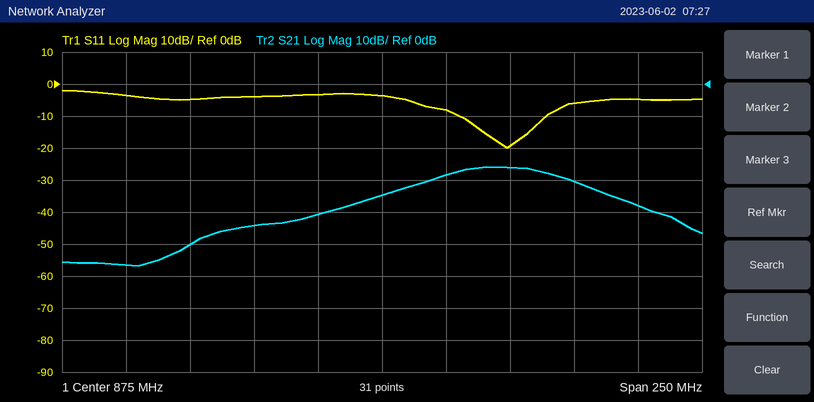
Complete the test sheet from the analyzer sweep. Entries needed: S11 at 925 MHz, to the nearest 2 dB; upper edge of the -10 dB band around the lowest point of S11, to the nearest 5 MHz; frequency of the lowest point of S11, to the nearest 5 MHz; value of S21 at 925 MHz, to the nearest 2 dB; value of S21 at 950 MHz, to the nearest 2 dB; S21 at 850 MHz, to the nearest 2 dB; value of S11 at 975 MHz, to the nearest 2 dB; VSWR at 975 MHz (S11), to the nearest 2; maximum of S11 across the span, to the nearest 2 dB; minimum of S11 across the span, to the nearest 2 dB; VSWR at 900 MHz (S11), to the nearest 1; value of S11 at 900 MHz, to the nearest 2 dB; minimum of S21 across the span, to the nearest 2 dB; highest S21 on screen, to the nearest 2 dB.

-20 dB
940 MHz
925 MHz
-26 dB
-30 dB
-40 dB
-4 dB
4
-2 dB
-20 dB
2
-8 dB
-56 dB
-26 dB
